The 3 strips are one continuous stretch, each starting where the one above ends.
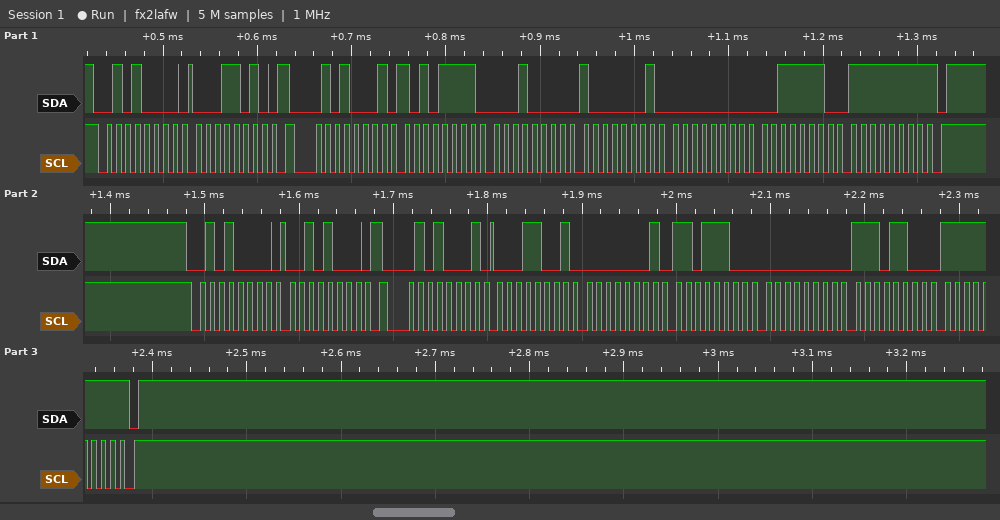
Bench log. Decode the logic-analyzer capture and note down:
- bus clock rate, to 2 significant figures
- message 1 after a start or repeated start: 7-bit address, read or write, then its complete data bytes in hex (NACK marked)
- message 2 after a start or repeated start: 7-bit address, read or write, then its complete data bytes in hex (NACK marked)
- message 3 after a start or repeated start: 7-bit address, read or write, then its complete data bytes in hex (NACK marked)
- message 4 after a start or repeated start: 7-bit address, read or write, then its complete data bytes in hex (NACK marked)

100 kHz
0x28 write: 1A
0x28 read: AF 10 81 00 3E FF NACK
0x28 write: 28
0x28 read: 19 01 DC 00 EC FF NACK
